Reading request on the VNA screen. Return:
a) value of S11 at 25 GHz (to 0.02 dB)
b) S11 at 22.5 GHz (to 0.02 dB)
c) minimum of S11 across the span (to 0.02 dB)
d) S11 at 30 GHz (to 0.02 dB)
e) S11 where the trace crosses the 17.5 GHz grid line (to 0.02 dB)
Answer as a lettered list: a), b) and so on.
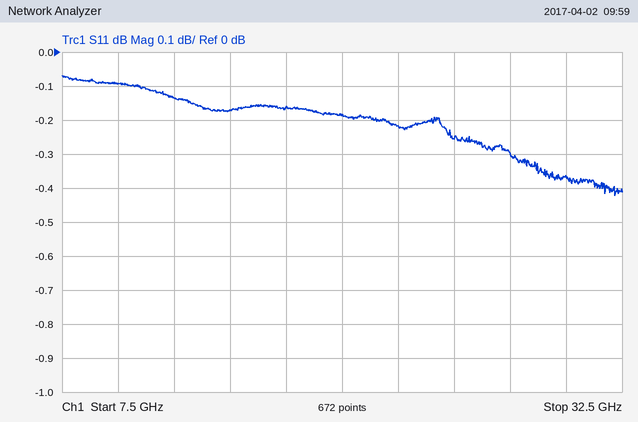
a) -0.26 dB
b) -0.22 dB
c) -0.42 dB
d) -0.36 dB
e) -0.16 dB
